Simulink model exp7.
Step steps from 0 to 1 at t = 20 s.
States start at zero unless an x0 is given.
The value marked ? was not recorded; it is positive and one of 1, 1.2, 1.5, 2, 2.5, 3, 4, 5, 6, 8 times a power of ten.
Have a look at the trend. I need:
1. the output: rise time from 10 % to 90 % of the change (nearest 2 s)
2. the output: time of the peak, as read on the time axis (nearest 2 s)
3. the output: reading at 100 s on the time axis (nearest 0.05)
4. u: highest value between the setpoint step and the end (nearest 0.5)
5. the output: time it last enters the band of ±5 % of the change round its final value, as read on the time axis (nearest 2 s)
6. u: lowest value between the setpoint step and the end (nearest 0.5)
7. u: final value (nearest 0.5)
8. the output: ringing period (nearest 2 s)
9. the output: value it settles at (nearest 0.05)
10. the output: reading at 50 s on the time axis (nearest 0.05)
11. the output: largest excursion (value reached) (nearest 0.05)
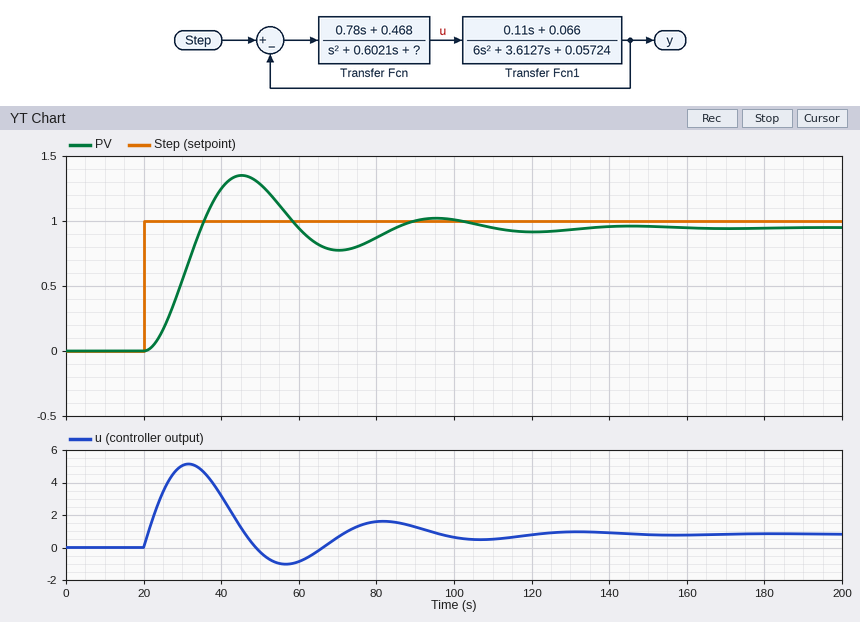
10 s
46 s
1.00
5.0
102 s
-1.0
1.0
50 s
0.95
1.30
1.35
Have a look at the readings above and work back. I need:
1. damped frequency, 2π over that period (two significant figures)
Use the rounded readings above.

0.13 rad/s
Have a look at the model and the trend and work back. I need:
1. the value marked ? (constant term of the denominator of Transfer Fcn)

0.03
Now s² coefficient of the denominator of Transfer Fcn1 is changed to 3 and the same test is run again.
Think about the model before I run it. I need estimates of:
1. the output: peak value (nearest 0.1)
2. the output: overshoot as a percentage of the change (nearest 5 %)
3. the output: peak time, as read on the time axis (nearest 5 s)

1.3
35 %
45 s
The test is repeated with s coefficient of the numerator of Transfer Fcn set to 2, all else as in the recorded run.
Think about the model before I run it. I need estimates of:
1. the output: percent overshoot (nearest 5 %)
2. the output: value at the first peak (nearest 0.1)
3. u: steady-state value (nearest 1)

25 %
1.2
1
